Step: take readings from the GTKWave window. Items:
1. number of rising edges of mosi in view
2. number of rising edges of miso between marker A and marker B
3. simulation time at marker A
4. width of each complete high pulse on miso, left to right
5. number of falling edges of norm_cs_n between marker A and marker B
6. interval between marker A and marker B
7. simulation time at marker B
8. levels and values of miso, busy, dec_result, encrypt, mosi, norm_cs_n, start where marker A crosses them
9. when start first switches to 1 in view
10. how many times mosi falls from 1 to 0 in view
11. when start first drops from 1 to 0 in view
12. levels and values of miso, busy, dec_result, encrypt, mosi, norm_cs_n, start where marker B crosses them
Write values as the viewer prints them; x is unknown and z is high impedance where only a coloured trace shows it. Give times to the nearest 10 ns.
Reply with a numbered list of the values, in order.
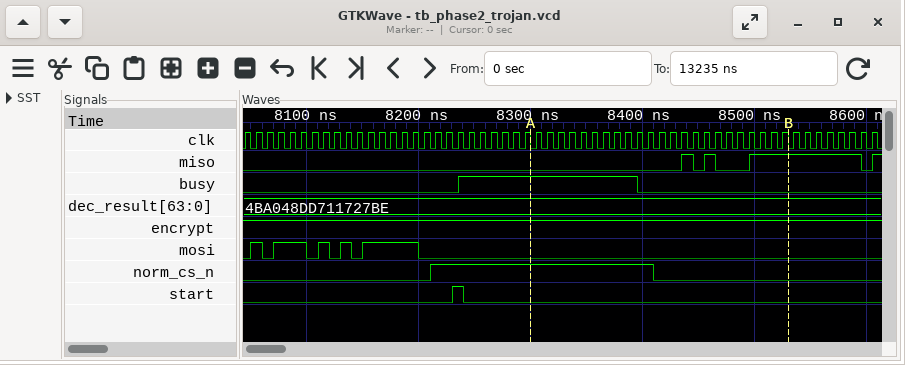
1. 5
2. 3
3. 8300 ns
4. 10 ns, 10 ns, 100 ns
5. 1
6. 230 ns
7. 8530 ns
8. miso=0, busy=1, dec_result=4BA048DD711727BE, encrypt=1, mosi=0, norm_cs_n=1, start=0
9. 8230 ns
10. 5
11. 8240 ns
12. miso=1, busy=0, dec_result=4BA048DD711727BE, encrypt=1, mosi=0, norm_cs_n=0, start=0
